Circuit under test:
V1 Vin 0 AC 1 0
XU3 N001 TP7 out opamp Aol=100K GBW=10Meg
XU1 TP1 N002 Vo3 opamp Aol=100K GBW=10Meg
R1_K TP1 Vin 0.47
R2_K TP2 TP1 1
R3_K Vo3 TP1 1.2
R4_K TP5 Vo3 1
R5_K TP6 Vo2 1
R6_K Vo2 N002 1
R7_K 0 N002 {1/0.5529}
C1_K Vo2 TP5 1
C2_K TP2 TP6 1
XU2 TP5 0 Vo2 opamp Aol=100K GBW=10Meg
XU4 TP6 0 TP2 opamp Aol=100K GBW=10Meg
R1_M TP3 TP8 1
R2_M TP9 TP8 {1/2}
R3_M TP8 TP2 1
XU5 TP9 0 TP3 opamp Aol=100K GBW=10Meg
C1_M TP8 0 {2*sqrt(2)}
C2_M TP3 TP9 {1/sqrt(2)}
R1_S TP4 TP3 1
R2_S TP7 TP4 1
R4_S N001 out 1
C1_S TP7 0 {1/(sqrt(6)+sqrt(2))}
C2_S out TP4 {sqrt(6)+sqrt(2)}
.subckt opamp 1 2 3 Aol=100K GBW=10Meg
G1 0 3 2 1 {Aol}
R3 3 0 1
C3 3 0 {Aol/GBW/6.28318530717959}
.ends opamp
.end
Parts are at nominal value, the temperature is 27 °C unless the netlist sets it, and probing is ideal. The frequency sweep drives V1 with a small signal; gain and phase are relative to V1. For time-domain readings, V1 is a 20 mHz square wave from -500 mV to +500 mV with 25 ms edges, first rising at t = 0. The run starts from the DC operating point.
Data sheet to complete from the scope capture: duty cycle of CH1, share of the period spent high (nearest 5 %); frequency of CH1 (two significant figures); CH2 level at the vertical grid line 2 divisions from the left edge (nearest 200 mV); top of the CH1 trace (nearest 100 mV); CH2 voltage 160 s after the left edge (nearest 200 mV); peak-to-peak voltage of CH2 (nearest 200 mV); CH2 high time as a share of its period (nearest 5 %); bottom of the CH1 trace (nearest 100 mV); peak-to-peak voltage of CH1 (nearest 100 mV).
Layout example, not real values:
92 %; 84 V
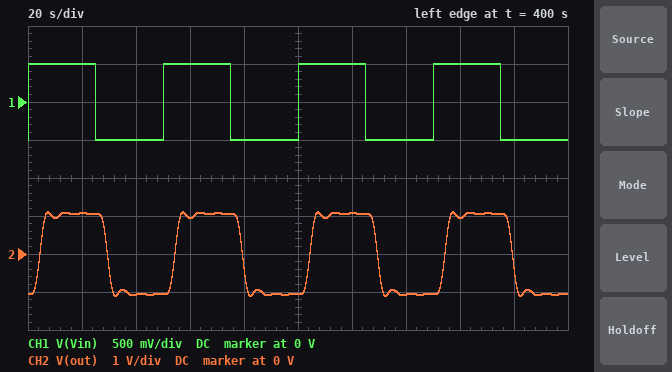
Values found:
50 %; 20 mHz; -1.0 V; 500 mV; 1.0 V; 2.2 V; 50 %; -500 mV; 1.0 V
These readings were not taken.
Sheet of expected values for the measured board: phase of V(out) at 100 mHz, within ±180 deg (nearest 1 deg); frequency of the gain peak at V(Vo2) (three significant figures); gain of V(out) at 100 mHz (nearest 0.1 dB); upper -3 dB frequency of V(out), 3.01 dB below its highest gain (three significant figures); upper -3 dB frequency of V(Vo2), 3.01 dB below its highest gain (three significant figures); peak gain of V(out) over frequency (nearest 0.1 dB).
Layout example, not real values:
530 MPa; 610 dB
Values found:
-151 deg; 174 mHz; 4.4 dB; 135 mHz; 543 mHz; 6.6 dB
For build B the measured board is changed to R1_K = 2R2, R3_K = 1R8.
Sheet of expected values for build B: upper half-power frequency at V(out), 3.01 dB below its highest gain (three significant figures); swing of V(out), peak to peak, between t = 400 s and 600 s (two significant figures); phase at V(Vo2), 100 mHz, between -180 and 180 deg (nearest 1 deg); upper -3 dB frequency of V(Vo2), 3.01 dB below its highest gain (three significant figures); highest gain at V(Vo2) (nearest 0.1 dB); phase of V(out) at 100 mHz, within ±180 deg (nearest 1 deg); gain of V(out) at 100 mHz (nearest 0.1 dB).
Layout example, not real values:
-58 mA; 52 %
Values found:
165 mHz; 680 mV; 44 deg; 468 mHz; -9.1 dB; -130 deg; -5.3 dB
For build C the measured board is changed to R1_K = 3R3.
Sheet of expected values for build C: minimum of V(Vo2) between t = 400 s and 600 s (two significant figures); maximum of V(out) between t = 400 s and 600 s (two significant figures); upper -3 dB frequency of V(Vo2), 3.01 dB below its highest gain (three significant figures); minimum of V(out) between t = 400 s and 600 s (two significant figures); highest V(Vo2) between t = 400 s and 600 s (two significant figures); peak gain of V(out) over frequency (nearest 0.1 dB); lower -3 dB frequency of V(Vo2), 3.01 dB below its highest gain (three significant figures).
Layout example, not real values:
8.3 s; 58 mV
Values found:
-150 mV; 230 mV; 350 mHz; -230 mV; 150 mV; -8.2 dB; 86.9 mHz
